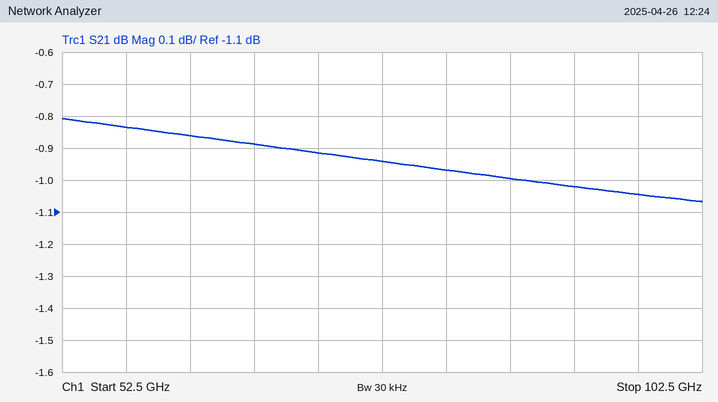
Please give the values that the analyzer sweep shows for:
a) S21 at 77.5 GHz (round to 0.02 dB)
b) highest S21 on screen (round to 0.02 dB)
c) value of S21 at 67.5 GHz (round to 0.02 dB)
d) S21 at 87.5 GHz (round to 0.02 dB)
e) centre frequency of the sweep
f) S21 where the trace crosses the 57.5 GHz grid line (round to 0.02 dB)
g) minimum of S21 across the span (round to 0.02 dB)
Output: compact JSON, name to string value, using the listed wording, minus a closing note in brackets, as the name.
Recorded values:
{"S21 at 77.5 GHz": "-0.94 dB", "highest S21 on screen": "-0.80 dB", "value of S21 at 67.5 GHz": "-0.88 dB", "S21 at 87.5 GHz": "-1.00 dB", "centre frequency of the sweep": "77.5 GHz", "S21 where the trace crosses the 57.5 GHz grid line": "-0.84 dB", "minimum of S21 across the span": "-1.06 dB"}
